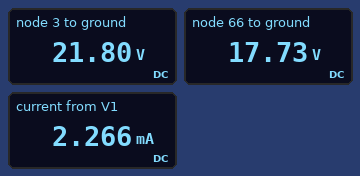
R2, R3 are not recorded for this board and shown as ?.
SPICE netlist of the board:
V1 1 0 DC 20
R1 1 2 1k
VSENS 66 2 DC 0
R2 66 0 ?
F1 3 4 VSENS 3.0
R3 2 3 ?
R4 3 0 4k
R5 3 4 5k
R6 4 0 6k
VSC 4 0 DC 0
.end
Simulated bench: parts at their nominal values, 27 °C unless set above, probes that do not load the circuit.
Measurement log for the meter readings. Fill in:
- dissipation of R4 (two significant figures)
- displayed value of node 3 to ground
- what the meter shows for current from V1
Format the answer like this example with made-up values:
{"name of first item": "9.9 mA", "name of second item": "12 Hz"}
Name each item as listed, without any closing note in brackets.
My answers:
{"dissipation of R4": "120 mW", "displayed value of node 3 to ground": "21.80 V", "what the meter shows for current from V1": "2.266 mA"}
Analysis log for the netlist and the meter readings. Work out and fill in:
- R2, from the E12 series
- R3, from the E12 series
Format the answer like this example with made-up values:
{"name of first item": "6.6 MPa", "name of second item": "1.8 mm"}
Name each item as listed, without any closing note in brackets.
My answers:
{"R2, from the E12 series": "4.7 kΩ", "R3, from the E12 series": "2.7 kΩ"}
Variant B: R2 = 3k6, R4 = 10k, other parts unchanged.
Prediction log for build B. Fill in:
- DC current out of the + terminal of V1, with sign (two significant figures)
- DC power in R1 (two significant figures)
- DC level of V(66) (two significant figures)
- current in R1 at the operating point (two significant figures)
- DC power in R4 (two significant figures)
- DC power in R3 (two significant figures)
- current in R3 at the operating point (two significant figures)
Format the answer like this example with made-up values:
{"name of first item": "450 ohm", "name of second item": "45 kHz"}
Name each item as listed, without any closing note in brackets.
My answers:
{"DC current out of the + terminal of V1, with sign": "-340 µA", "DC power in R1": "120 µW", "DC level of V(66)": "20 V", "current in R1 at the operating point": "340 µA", "DC power in R4": "130 mW", "DC power in R3": "97 mW", "current in R3 at the operating point": "6.0 mA"}
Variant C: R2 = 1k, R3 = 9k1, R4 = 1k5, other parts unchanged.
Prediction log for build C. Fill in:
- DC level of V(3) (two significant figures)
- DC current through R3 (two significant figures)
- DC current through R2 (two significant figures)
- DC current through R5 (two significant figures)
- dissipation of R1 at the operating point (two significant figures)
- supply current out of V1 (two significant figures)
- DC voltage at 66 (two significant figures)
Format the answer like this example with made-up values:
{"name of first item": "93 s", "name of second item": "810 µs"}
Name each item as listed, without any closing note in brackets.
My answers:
{"DC level of V(3)": "36 V", "DC current through R3": "2.7 mA", "DC current through R2": "11 mA", "DC current through R5": "7.2 mA", "dissipation of R1 at the operating point": "75 mW", "supply current out of V1": "8.6 mA", "DC voltage at 66": "11 V"}
